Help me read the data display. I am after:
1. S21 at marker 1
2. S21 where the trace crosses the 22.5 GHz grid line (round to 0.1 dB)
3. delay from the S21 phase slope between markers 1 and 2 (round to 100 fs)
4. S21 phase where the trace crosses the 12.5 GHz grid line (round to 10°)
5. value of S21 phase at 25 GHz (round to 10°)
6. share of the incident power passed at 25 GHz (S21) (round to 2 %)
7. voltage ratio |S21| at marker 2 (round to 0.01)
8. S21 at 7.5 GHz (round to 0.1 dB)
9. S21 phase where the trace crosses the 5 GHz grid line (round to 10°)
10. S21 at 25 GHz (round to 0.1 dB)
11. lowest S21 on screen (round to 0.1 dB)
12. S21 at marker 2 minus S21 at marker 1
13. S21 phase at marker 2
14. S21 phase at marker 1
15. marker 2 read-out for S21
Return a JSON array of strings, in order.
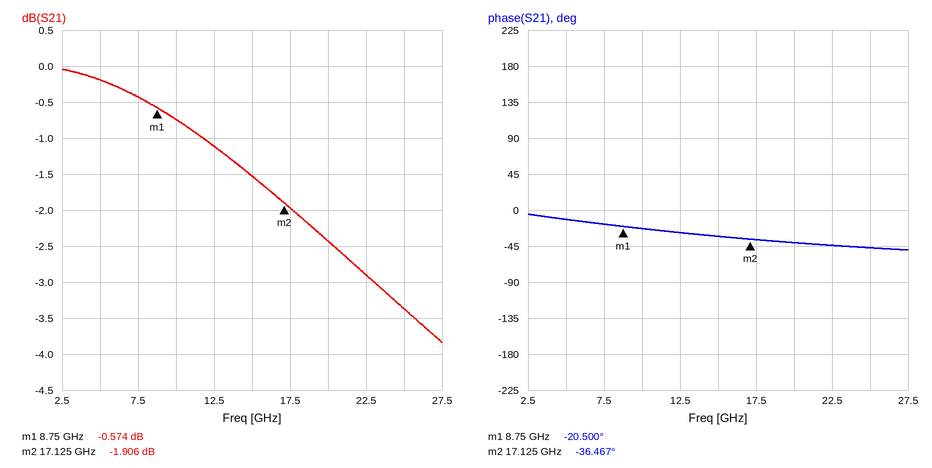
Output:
["-0.574 dB", "-2.9 dB", "5.3 ps", "-30°", "-50°", "46 %", "0.80", "-0.4 dB", "-10°", "-3.4 dB", "-3.8 dB", "-1.332 dB", "-36.467°", "-20.500°", "-1.906 dB"]
